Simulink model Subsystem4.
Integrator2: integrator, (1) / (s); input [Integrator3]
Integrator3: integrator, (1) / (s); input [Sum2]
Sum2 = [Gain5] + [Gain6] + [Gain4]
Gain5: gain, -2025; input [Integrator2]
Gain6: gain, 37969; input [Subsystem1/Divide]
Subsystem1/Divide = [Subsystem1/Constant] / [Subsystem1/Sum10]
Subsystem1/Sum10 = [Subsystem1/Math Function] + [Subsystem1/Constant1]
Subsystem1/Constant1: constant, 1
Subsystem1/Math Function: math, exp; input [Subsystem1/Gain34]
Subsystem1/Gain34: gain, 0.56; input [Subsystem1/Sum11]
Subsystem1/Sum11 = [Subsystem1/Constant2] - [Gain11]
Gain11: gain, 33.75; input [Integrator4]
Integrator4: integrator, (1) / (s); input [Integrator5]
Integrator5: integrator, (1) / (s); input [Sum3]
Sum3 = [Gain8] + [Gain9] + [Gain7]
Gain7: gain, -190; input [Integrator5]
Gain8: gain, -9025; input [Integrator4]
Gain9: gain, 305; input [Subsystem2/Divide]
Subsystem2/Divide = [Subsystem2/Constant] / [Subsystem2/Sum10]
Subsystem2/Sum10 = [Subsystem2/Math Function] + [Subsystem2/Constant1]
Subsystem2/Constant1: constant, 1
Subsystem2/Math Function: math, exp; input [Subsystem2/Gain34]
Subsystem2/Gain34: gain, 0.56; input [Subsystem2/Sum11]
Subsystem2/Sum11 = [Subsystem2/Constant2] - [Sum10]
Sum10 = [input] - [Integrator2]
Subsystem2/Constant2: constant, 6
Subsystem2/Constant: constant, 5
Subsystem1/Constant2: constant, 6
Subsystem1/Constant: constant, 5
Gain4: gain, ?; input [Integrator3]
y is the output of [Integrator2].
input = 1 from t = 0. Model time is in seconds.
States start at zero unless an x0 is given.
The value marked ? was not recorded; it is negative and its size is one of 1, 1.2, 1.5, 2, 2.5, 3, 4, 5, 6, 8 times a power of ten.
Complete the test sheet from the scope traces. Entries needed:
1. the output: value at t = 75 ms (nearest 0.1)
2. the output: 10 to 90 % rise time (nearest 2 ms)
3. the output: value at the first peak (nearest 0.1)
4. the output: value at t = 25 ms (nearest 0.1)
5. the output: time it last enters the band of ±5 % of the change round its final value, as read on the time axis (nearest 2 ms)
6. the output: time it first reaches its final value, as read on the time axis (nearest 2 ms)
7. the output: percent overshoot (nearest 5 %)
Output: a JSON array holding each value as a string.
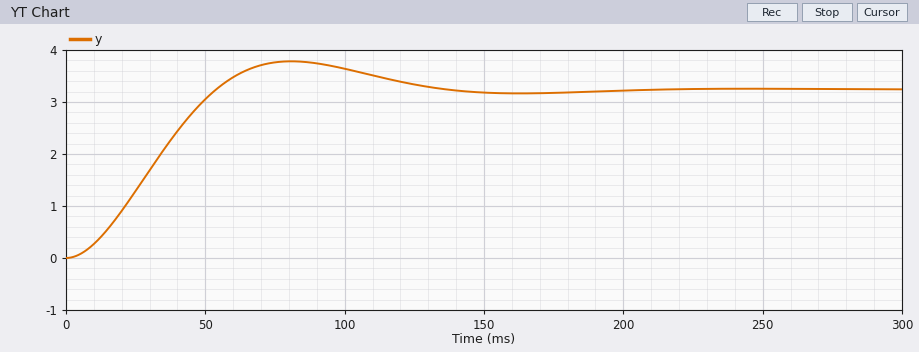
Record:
["3.8", "36 ms", "3.8", "1.3", "118 ms", "54 ms", "15 %"]
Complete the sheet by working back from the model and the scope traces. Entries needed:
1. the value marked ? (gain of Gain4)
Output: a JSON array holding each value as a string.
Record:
["-50"]
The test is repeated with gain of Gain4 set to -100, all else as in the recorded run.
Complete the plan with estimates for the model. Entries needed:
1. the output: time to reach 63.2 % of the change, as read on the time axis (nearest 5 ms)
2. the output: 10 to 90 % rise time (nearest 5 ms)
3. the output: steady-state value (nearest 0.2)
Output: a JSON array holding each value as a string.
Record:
["50 ms", "75 ms", "3.2"]
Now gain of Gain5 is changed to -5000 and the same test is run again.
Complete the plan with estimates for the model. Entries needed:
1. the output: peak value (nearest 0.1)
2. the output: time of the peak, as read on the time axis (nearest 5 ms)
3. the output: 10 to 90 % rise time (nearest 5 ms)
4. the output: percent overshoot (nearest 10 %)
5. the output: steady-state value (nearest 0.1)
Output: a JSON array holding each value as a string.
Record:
["1.8", "50 ms", "20 ms", "30 %", "1.4"]
